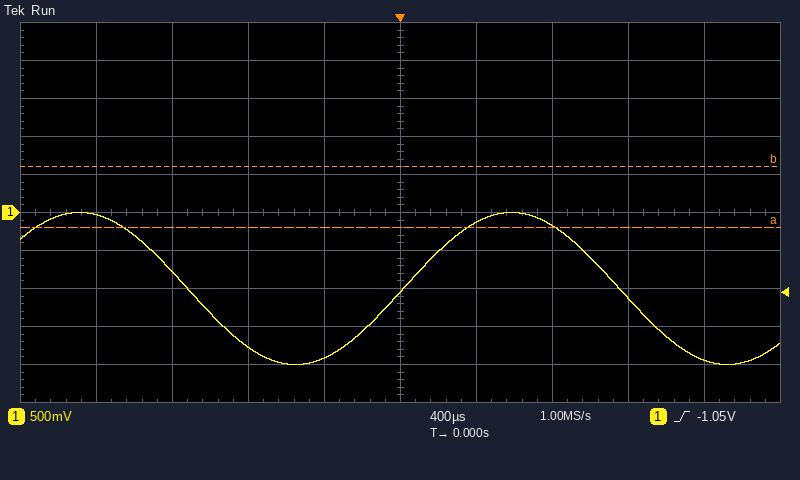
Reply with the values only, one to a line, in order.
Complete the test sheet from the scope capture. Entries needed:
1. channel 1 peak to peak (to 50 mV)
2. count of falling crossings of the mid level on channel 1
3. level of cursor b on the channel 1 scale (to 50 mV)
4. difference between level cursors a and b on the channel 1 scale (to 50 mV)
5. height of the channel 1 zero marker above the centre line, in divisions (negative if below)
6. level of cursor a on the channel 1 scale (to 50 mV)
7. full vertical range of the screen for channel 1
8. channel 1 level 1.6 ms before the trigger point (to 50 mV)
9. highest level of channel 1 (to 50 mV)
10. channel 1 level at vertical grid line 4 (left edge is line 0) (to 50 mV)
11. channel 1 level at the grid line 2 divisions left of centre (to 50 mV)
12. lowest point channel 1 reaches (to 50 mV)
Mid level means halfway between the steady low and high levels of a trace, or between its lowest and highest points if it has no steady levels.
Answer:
2.00 V
2
600 mV
800 mV
0.0 div
-200 mV
5 V
-50 mV
0 mV
-1.90 V
-1.75 V
-2.00 V
